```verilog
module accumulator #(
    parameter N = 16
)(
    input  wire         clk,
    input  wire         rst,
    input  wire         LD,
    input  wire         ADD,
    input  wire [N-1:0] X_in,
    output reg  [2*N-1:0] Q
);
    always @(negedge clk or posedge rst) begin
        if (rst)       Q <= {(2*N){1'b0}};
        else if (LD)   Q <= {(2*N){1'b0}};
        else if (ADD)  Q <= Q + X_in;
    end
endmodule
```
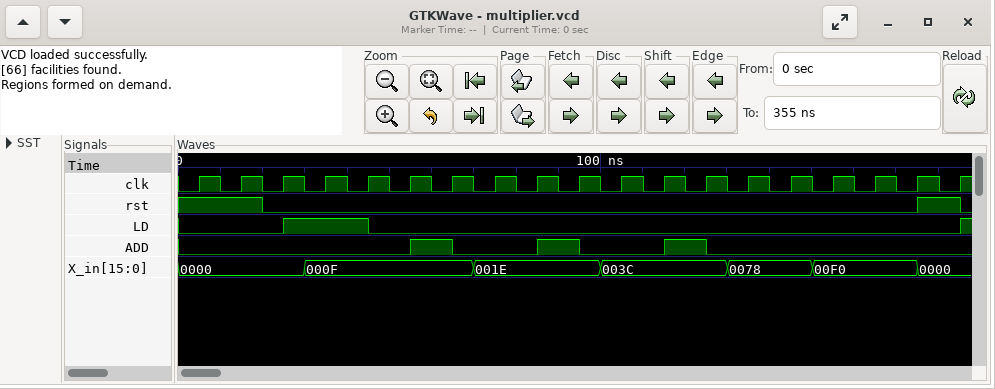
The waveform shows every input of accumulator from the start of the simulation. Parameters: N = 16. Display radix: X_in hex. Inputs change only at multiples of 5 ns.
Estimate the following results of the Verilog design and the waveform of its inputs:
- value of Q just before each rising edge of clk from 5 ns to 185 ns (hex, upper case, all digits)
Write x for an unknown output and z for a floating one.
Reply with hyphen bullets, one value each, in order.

- 00000000, 00000000, 00000000, 00000000, 00000000, 00000000, 0000000F, 0000000F, 0000000F, 0000002D, 0000002D, 0000002D, 00000069, 00000069, 00000069, 00000069, 00000069, 00000069, 00000000
